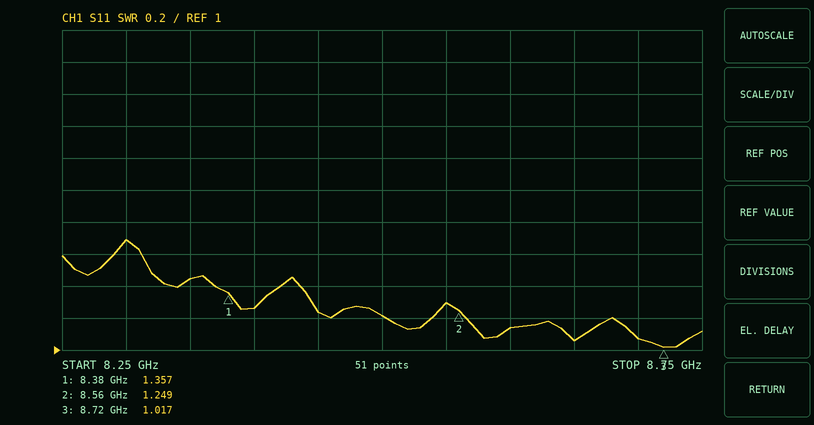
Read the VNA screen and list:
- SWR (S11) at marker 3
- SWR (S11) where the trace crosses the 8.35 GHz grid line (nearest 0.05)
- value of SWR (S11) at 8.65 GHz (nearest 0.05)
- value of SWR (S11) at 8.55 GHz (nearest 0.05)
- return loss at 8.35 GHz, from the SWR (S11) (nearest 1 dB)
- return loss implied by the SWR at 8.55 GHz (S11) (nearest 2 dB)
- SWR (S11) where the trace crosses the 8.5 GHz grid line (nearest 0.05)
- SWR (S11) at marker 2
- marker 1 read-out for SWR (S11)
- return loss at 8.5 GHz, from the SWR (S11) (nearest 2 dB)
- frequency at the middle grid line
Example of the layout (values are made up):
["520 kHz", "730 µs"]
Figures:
["1.017", "1.45", "1.05", "1.30", "15 dB", "18 dB", "1.20", "1.249", "1.357", "20 dB", "8.5 GHz"]
